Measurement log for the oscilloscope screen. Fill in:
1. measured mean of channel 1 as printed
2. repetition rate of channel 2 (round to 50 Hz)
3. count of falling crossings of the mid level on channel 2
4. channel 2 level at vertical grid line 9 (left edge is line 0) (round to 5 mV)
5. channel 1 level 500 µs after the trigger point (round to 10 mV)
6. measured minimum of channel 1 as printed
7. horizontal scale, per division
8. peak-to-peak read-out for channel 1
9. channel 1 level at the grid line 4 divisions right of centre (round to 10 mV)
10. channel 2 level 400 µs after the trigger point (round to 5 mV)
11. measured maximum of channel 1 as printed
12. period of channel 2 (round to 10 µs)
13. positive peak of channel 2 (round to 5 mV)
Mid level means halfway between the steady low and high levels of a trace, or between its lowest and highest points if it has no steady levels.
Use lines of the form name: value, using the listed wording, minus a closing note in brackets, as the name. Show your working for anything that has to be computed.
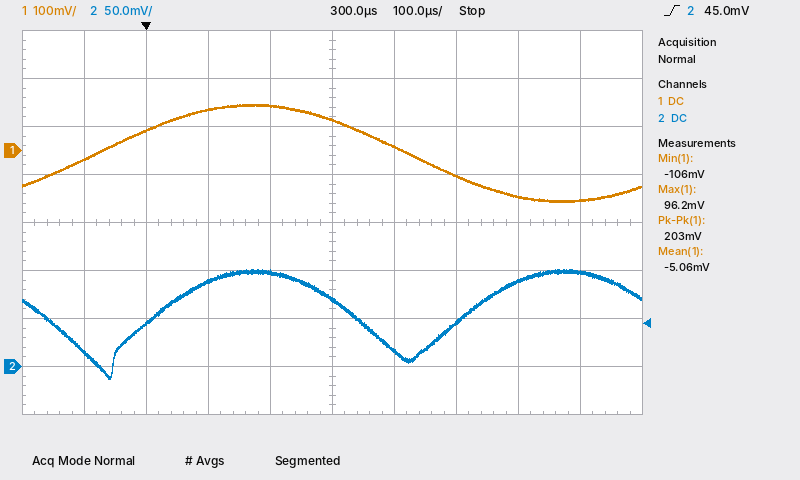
measured mean of channel 1 as printed: -5.06 mV
repetition rate of channel 2: 1 / 500 µs ≈ 2.00 kHz
count of falling crossings of the mid level on channel 2: 2
channel 2 level at vertical grid line 9 (left edge is line 0): 100 mV
channel 1 level 500 µs after the trigger point: -50 mV
measured minimum of channel 1 as printed: -106 mV
horizontal scale, per division: 100 µs
peak-to-peak read-out for channel 1: 203 mV
channel 1 level at the grid line 4 divisions right of centre: -100 mV
channel 2 level 400 µs after the trigger point: 15 mV
measured maximum of channel 1 as printed: 96.2 mV
period of channel 2: 500 µs
positive peak of channel 2: 100 mV
